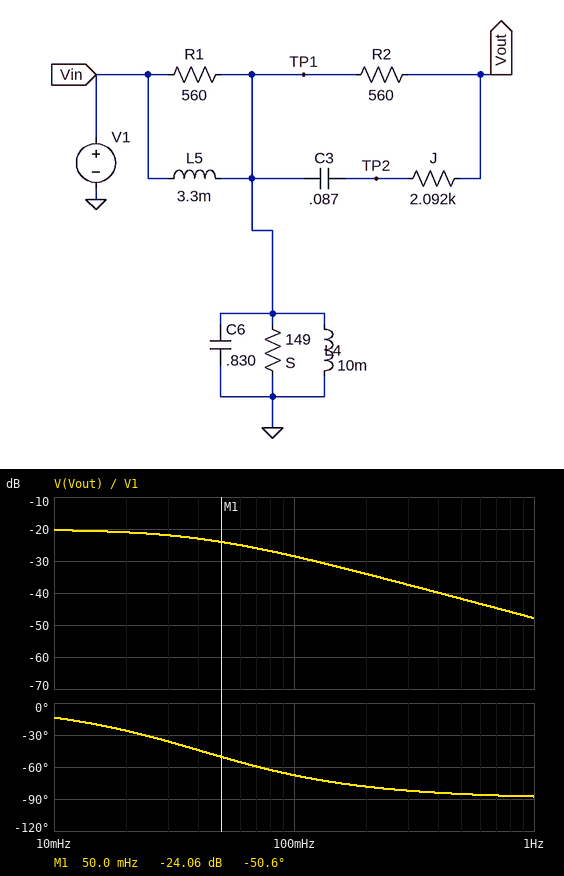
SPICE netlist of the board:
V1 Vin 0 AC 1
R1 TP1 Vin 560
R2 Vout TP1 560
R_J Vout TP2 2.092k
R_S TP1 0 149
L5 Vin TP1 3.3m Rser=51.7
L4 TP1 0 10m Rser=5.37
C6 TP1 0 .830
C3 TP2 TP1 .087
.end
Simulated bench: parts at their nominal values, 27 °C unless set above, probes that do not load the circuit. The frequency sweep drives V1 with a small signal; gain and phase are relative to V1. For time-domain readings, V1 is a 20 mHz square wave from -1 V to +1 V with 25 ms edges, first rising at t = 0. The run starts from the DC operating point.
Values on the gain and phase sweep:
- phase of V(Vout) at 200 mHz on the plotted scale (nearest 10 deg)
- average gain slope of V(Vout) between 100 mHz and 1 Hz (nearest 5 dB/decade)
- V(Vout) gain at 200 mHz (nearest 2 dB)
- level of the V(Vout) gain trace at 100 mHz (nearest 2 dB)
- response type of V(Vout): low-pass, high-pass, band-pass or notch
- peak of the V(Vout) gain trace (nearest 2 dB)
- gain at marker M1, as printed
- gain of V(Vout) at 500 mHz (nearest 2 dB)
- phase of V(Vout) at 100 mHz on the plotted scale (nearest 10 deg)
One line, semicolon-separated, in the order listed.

-80 deg; -20 dB/decade; -34 dB; -28 dB; low-pass; -20 dB; -24.06 dB; -42 dB; -70 deg
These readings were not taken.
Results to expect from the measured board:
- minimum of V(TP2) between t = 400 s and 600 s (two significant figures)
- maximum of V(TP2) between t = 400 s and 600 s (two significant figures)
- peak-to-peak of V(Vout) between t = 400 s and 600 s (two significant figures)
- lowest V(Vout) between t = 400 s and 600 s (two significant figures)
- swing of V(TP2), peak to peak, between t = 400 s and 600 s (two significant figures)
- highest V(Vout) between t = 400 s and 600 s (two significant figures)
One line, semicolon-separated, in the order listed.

-98 mV; 98 mV; 200 mV; -98 mV; 200 mV; 98 mV
